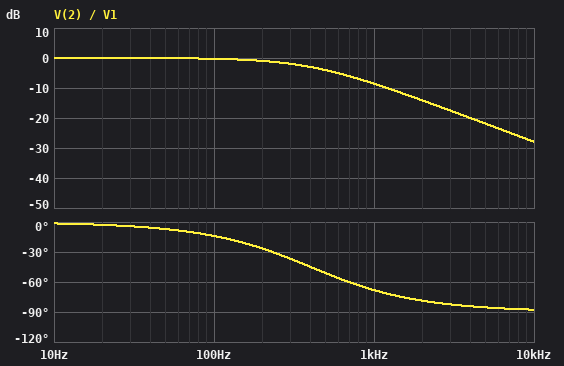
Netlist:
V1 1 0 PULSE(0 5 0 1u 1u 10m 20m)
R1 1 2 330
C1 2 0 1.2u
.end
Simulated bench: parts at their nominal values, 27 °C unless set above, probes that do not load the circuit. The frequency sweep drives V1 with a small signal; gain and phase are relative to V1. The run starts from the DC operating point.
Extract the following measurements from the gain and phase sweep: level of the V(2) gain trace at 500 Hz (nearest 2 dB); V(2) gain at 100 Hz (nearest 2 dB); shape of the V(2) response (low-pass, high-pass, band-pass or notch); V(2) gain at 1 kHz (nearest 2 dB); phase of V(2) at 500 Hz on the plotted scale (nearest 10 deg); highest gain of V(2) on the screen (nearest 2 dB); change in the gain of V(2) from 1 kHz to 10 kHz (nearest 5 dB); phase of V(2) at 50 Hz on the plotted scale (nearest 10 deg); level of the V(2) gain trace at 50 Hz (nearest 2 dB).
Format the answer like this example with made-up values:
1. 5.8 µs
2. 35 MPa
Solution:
1. -4 dB
2. 0 dB
3. low-pass
4. -8 dB
5. -50 deg
6. 0 dB
7. -20 dB
8. -10 deg
9. 0 dB
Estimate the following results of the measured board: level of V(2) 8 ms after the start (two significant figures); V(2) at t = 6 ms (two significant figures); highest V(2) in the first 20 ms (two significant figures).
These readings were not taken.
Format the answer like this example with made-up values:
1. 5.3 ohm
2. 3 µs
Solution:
1. 5.0 V
2. 5.0 V
3. 5.0 V
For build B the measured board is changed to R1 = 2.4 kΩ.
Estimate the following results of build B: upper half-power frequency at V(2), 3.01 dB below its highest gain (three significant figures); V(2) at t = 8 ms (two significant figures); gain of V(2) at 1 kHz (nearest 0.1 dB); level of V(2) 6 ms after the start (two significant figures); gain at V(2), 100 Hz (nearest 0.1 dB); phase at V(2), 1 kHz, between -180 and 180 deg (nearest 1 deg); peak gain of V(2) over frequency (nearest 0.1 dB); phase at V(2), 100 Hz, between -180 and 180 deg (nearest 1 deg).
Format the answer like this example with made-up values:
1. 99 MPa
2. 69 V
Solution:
1. 55.3 Hz
2. 4.7 V
3. -25.2 dB
4. 4.4 V
5. -6.3 dB
6. -87 deg
7. 0 dB
8. -61 deg
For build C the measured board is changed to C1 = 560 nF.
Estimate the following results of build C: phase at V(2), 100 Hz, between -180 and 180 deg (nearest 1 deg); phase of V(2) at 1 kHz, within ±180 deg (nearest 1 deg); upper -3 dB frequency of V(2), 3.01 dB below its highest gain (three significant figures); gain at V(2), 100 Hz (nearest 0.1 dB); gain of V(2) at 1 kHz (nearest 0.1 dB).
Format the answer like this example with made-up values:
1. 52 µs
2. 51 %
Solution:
1. -7 deg
2. -49 deg
3. 861 Hz
4. -0.1 dB
5. -3.7 dB
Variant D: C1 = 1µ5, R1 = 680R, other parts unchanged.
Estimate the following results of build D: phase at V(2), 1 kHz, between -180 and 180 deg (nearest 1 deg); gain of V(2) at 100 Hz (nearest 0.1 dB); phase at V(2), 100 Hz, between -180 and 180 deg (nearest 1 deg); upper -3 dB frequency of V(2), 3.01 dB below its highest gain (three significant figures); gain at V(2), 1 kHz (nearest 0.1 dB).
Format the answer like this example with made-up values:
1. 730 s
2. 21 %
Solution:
1. -81 deg
2. -1.5 dB
3. -33 deg
4. 156 Hz
5. -16.2 dB
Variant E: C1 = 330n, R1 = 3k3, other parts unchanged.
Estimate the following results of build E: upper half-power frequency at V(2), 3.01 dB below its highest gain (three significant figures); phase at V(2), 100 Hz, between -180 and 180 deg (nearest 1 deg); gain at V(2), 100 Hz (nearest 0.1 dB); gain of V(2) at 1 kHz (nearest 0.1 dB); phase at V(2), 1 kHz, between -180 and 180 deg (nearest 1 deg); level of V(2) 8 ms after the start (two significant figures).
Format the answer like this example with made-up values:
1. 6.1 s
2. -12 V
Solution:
1. 146 Hz
2. -34 deg
3. -1.7 dB
4. -16.8 dB
5. -82 deg
6. 5.0 V
